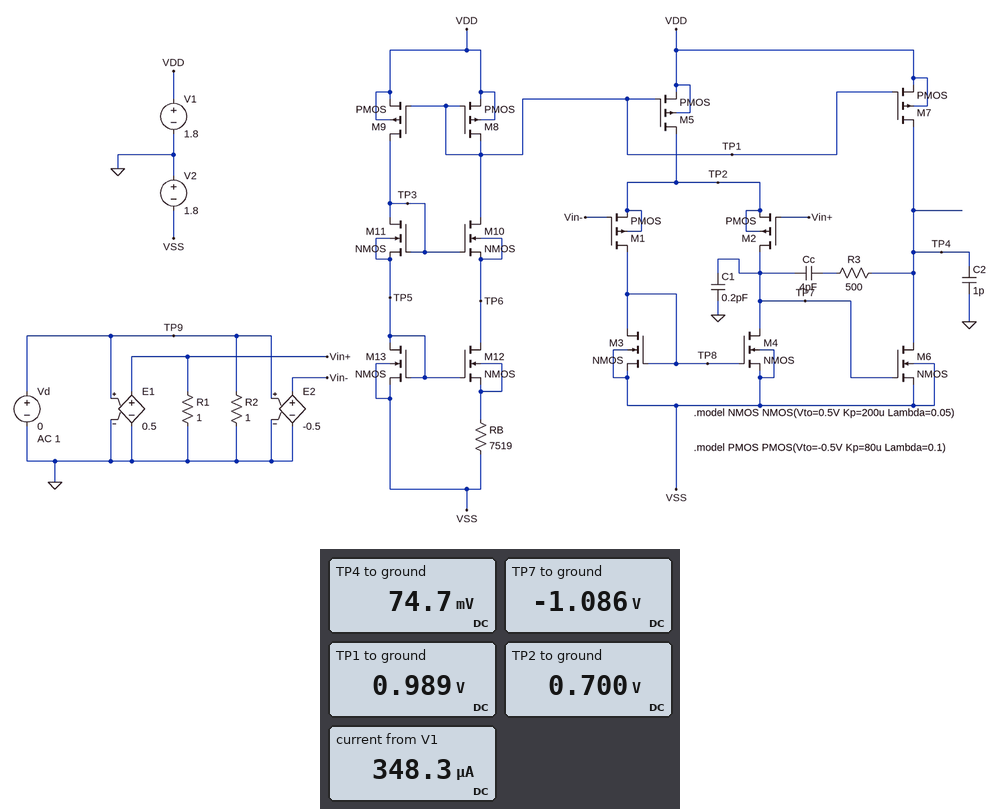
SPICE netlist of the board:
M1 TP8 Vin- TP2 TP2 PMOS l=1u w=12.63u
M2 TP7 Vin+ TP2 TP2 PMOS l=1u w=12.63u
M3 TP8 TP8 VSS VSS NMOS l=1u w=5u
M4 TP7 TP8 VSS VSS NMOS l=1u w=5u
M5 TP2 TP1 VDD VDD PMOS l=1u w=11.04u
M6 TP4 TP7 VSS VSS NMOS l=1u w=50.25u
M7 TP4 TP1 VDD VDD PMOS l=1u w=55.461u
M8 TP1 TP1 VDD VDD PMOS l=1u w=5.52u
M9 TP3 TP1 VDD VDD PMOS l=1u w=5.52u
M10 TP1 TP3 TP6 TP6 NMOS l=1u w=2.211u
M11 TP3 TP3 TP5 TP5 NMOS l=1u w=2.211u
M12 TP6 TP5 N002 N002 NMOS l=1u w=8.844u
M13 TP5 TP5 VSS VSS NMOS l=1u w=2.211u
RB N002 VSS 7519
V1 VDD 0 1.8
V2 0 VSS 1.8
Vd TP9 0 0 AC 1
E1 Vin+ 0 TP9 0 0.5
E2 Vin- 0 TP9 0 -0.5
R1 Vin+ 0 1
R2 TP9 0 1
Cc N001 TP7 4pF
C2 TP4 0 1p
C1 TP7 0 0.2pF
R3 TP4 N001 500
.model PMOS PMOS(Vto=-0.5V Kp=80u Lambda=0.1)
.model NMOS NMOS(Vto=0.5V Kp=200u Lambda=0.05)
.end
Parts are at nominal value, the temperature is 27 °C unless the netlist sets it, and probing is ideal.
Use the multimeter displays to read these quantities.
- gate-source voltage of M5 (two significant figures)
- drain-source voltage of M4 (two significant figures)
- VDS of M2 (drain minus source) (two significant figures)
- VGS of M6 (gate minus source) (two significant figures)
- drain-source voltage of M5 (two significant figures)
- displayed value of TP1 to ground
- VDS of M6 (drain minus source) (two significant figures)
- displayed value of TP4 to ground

-810 mV
710 mV
-1.8 V
710 mV
-1.1 V
0.989 V
1.9 V
74.7 mV
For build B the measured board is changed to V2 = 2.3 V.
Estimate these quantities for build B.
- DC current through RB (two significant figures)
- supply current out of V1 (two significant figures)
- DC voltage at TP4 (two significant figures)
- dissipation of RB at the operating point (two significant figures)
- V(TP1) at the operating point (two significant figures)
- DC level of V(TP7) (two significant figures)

25 µA
380 µA
-95 mV
4.6 µW
980 mV
-1.6 V
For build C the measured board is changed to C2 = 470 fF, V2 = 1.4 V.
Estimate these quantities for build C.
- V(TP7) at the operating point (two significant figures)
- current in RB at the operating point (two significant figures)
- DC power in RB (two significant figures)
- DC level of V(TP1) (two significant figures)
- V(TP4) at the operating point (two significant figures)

-690 mV
22 µA
3.6 µW
1.0 V
210 mV
